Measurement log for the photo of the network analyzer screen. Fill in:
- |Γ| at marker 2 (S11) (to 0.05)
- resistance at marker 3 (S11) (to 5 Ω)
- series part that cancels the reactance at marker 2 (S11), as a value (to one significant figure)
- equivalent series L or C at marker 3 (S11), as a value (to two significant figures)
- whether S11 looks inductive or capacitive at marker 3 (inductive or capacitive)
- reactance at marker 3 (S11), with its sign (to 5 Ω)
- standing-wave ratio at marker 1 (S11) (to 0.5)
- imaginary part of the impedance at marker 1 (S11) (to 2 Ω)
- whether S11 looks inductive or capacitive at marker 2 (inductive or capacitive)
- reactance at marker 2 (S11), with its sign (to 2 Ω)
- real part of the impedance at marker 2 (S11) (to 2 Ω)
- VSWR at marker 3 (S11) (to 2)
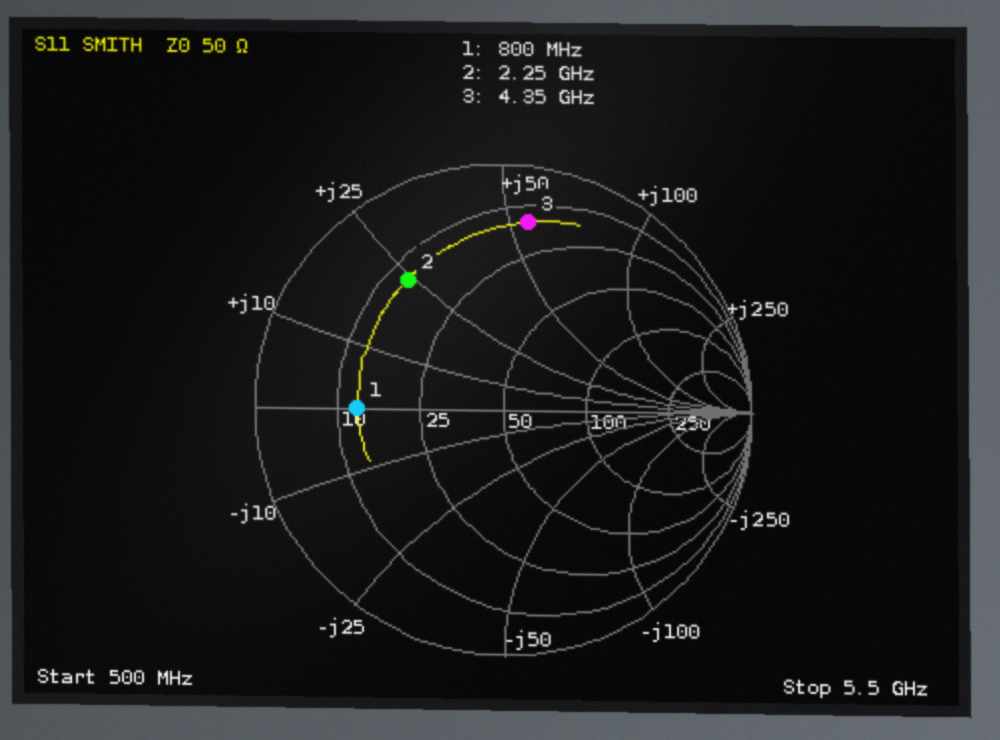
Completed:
0.65
15 Ω
3 pF
2.0 nH
inductive
+55 Ω
4.0
0 Ω
inductive
+24 Ω
14 Ω
8
